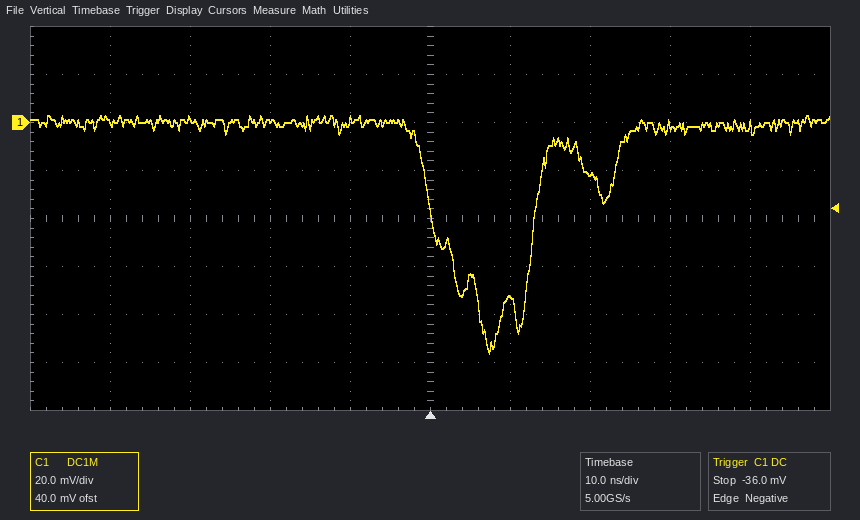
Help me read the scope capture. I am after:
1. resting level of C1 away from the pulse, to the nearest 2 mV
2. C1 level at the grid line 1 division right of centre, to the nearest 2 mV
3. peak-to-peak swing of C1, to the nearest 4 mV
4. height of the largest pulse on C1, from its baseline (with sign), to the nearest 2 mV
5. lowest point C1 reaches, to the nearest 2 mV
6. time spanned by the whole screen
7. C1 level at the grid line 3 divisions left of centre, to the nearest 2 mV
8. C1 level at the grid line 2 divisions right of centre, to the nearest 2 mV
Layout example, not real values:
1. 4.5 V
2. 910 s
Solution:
1. 0 mV
2. -74 mV
3. 100 mV
4. -96 mV
5. -96 mV
6. 100 ns
7. 2 mV
8. -22 mV
